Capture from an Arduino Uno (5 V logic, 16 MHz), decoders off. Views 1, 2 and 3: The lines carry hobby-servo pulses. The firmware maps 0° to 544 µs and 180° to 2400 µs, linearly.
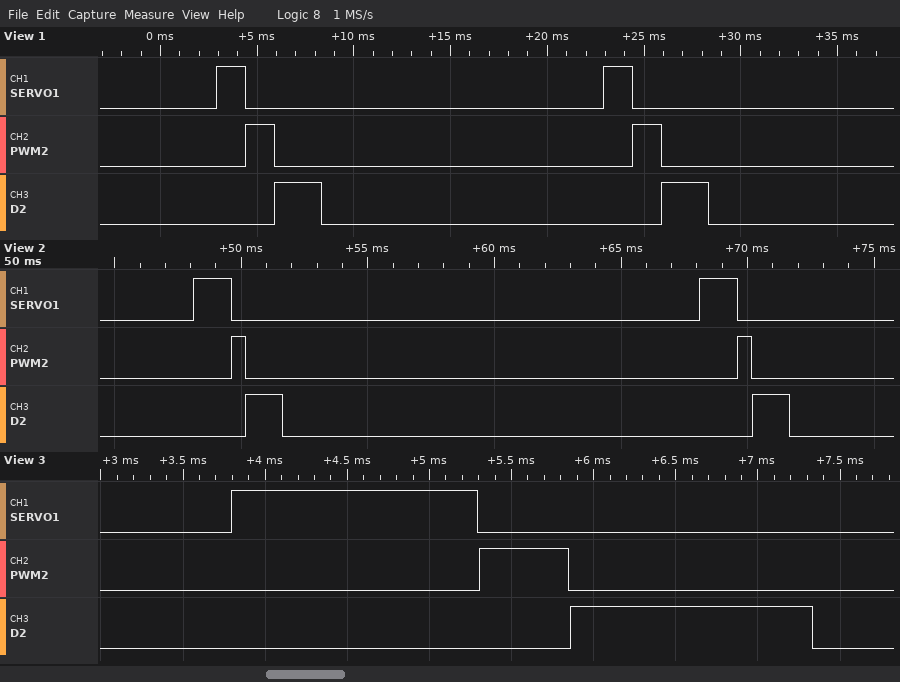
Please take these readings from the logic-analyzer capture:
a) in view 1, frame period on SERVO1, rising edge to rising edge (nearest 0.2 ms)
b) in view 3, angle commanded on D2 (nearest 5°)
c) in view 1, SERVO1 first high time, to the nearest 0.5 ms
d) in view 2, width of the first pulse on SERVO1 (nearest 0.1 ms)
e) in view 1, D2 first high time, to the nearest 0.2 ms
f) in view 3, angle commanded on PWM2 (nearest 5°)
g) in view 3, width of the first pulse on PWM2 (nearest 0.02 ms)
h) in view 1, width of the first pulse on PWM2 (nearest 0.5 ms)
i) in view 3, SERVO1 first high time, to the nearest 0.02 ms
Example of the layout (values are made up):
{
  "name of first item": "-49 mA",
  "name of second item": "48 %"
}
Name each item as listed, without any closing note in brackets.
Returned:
{
  "in view 1, frame period on SERVO1, rising edge to rising edge": "20.0 ms",
  "in view 3, angle commanded on D2": "90°",
  "in view 1, SERVO1 first high time, to the nearest 0.5 ms": "1.5 ms",
  "in view 2, width of the first pulse on SERVO1": "1.5 ms",
  "in view 1, D2 first high time, to the nearest 0.2 ms": "2.4 ms",
  "in view 3, angle commanded on PWM2": "0°",
  "in view 3, width of the first pulse on PWM2": "0.54 ms",
  "in view 1, width of the first pulse on PWM2": "1.5 ms",
  "in view 3, SERVO1 first high time, to the nearest 0.02 ms": "1.50 ms"
}
